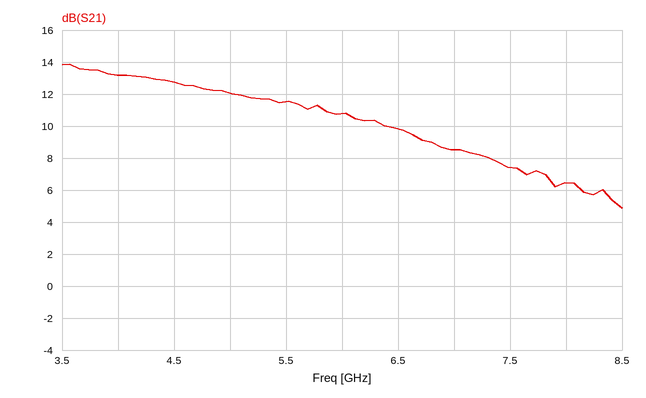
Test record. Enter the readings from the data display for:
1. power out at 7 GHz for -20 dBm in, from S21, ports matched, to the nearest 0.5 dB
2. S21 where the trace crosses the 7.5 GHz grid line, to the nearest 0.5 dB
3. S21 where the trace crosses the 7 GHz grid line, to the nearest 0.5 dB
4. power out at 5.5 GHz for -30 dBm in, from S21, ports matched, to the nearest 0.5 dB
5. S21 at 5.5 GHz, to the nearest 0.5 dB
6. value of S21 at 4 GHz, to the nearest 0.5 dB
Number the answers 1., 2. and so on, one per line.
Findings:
1. -11.5 dBm
2. 7.5 dB
3. 8.5 dB
4. -18.5 dBm
5. 11.5 dB
6. 13.0 dB
